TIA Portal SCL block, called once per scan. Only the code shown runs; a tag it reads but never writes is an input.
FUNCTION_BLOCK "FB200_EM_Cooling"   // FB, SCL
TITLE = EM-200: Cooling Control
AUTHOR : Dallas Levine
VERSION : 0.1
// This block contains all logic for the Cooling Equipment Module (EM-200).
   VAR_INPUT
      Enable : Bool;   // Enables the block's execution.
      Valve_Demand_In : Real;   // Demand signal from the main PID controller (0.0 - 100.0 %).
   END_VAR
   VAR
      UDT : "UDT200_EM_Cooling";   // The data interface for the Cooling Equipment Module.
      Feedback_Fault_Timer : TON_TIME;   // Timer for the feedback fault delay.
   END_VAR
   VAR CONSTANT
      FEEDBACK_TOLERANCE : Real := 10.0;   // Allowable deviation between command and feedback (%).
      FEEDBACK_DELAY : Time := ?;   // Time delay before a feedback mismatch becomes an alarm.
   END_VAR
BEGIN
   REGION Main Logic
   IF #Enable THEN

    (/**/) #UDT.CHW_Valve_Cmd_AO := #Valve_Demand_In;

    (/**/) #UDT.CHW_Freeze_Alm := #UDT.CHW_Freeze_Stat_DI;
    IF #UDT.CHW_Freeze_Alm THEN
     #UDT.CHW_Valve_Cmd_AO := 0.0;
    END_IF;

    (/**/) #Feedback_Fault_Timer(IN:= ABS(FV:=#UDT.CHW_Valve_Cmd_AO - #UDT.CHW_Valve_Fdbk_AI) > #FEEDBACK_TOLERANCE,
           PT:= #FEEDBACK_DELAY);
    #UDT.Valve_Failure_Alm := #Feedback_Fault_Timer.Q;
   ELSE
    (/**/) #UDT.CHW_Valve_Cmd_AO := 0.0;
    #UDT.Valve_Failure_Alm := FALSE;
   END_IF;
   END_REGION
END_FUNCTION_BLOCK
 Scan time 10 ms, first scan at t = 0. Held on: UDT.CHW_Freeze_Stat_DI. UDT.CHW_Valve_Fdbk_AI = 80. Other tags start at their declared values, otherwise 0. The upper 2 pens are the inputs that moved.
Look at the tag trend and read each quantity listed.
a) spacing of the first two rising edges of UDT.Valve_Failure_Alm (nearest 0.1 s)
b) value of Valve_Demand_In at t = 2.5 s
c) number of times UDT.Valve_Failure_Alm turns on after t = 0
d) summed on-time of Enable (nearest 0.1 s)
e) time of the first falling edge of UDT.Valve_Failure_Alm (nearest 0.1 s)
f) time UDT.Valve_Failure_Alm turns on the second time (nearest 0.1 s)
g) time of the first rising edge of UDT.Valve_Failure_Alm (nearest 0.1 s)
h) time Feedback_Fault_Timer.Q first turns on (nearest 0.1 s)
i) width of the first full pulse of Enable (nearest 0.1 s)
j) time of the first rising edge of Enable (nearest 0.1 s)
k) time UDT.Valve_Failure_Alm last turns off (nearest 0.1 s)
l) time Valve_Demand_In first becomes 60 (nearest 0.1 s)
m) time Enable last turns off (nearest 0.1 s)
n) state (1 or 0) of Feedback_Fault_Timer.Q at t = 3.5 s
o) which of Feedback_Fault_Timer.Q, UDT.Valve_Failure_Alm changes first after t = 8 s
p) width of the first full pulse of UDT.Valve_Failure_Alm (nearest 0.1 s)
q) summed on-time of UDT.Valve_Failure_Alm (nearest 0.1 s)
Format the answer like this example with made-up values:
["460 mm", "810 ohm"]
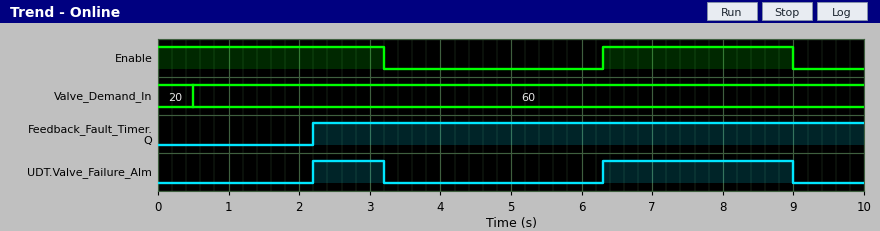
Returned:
["4.1 s", "60", "2", "5.9 s", "3.2 s", "6.3 s", "2.2 s", "2.2 s", "2.7 s", "6.3 s", "9.0 s", "0.5 s", "9.0 s", "1", "UDT.Valve_Failure_Alm", "1.0 s", "3.7 s"]
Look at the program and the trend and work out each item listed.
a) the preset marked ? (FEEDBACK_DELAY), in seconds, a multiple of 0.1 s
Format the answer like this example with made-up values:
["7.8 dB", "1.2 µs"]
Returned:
["2.2 s"]
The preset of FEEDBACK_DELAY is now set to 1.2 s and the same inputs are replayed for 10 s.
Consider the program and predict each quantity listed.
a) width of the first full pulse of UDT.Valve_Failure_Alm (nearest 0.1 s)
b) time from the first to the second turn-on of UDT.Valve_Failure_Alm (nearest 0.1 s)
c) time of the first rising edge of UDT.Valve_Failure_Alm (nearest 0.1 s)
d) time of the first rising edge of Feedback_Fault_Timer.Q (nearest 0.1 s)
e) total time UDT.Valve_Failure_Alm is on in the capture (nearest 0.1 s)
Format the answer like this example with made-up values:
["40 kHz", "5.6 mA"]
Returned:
["2.0 s", "5.1 s", "1.2 s", "1.2 s", "4.7 s"]
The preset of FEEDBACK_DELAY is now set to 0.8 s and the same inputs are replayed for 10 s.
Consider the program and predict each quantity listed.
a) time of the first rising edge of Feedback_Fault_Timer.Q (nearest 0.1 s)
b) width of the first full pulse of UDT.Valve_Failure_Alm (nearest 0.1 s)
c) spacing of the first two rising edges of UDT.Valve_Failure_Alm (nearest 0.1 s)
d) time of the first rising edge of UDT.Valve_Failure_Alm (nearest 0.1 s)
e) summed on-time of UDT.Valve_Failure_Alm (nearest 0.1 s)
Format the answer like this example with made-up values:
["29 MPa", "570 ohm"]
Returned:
["0.8 s", "2.4 s", "5.5 s", "0.8 s", "5.1 s"]
